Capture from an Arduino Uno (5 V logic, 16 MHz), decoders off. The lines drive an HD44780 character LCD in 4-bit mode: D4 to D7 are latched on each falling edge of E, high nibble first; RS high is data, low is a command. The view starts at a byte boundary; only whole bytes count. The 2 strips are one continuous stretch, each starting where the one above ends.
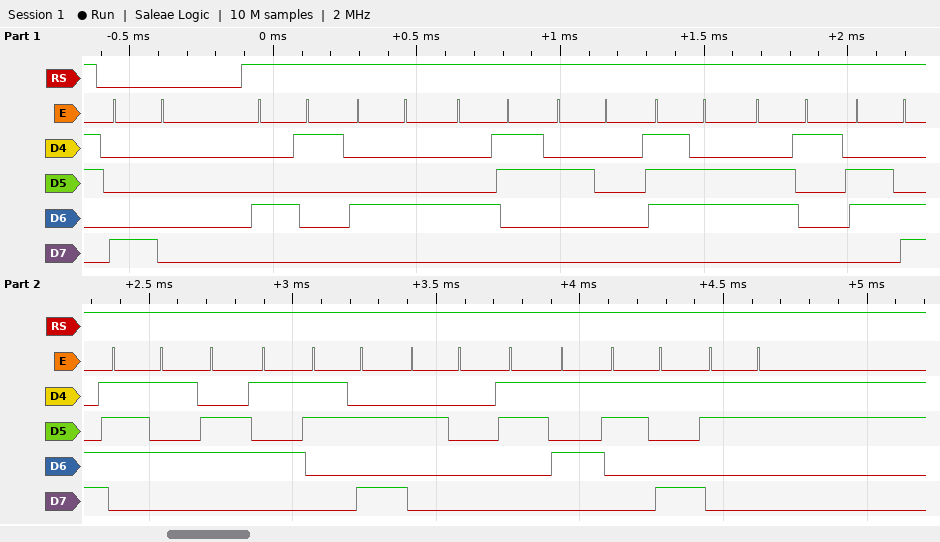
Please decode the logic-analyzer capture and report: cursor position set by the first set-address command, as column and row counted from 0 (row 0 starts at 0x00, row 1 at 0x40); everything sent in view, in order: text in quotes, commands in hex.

column 0, row 0
0x80 "ADC value: 593"
